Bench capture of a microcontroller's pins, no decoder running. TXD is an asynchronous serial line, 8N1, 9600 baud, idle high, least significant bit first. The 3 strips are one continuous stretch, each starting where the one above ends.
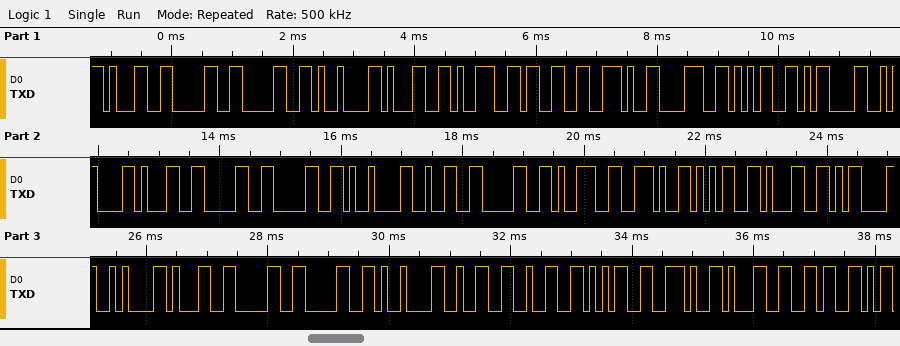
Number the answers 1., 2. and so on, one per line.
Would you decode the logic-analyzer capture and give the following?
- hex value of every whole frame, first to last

1. 31 30 30 09 31 39 33 2E 38 35 0D 0A 31 30 30 09 32 30 39 2E 35 31 0D 0A 31 30 30 09 32 32 35 2E 31 36
